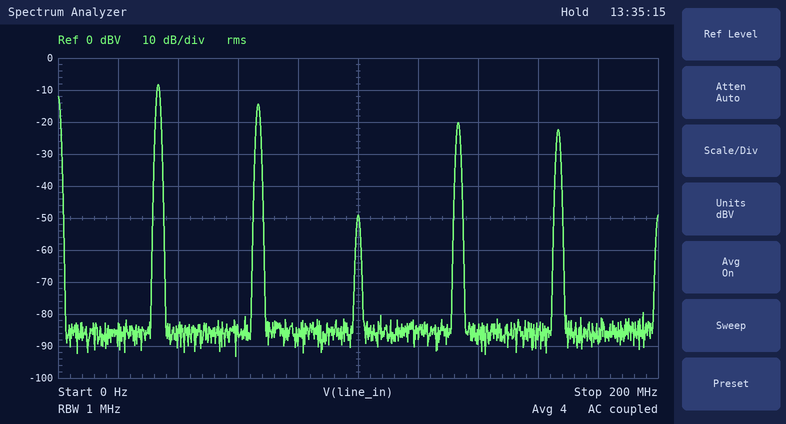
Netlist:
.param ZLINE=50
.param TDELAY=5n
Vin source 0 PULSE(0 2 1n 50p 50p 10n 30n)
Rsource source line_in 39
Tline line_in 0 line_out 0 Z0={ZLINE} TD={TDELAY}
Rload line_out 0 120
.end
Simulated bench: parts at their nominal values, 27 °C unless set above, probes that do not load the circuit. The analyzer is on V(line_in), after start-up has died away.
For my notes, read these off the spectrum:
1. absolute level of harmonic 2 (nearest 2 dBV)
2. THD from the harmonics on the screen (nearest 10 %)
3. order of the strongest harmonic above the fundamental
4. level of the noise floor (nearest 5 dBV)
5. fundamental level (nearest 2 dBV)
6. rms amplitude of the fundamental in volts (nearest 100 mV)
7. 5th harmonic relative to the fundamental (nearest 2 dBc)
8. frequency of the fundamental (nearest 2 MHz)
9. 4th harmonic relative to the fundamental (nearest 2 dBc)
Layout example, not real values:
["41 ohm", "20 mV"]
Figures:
["-14 dBV", "60 %", "2", "-85 dBV", "-8 dBV", "400 mV", "-14 dBc", "34 MHz", "-12 dBc"]
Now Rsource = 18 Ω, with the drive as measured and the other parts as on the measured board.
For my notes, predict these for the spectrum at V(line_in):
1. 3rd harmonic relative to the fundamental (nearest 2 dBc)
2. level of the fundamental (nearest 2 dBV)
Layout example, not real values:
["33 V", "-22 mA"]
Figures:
["-42 dBc", "-6 dBV"]
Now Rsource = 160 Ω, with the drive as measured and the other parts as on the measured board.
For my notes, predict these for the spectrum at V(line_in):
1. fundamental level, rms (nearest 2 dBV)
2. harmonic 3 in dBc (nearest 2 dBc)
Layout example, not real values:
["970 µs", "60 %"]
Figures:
["-16 dBV", "-36 dBc"]
